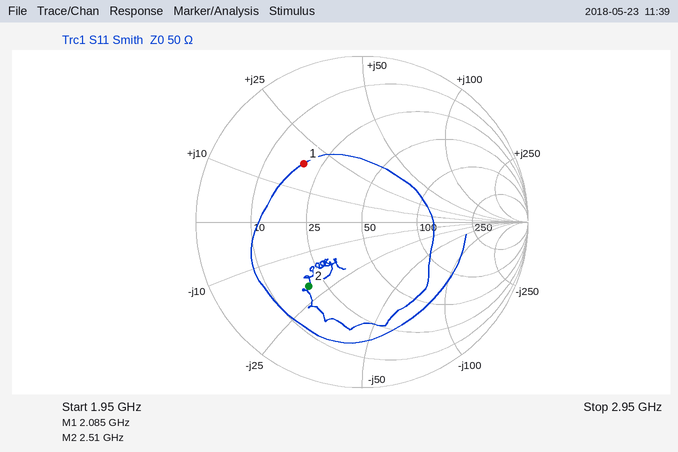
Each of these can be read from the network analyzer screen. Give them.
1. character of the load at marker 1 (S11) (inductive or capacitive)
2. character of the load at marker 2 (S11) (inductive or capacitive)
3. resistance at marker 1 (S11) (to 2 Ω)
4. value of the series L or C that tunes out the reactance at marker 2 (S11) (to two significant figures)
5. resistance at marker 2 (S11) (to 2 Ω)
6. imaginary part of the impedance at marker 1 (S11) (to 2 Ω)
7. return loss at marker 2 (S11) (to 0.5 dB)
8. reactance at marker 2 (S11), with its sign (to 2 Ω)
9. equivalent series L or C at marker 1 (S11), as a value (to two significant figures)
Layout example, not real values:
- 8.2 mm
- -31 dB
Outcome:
- inductive
- capacitive
- 20 Ω
- 1.3 nH
- 20 Ω
- +18 Ω
- 6.0 dB
- -20 Ω
- 1.4 nH
